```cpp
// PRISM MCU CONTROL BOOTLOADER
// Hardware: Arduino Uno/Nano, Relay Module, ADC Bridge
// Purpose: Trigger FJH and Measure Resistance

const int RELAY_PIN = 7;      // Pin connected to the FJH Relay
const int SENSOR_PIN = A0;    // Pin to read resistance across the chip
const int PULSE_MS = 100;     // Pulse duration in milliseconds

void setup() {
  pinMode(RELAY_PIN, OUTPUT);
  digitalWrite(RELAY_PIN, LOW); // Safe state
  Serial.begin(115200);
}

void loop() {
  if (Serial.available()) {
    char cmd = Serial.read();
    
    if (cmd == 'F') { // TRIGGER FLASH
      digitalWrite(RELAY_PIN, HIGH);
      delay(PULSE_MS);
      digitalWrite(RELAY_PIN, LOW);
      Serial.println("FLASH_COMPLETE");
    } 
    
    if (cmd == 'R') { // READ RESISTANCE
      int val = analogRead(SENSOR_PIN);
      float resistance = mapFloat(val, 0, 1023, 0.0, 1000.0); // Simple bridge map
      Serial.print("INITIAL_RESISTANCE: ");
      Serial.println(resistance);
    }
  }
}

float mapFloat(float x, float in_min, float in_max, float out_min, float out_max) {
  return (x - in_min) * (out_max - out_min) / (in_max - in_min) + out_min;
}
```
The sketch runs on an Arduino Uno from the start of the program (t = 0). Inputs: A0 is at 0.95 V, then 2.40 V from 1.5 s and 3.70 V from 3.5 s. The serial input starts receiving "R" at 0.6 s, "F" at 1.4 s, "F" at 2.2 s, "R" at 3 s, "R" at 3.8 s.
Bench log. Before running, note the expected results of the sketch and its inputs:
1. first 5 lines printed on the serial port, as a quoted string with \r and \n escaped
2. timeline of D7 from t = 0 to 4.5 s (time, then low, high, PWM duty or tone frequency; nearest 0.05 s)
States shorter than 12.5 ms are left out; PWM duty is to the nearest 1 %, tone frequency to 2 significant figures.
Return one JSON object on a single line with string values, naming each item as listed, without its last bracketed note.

{"first 5 lines printed on the serial port, as a quoted string with \\r and \\n escaped": "\"INITIAL_RESISTANCE: 189.64\\r\\nFLASH_COMPLETE\\r\\nFLASH_COMPLETE\\r\\nINITIAL_RESISTANCE: 479.96\\r\\nINITIAL_RESISTANCE: 739.98\\r\\n\"", "timeline of D7 from t = 0 to 4.5 s": "0 s low; 1.4 s high; 1.5 s low; 2.2 s high; 2.3 s low"}
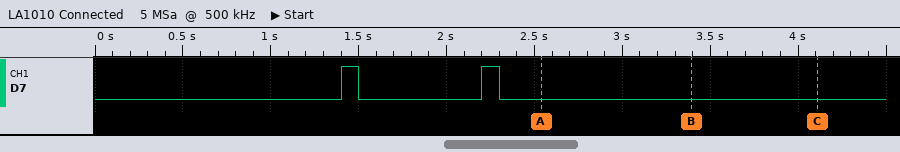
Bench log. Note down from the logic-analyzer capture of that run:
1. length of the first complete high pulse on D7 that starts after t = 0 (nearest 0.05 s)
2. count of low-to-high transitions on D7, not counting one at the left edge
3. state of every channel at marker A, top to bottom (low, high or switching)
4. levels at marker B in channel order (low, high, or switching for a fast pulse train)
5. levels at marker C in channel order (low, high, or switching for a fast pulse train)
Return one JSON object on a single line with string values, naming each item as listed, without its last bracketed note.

{"length of the first complete high pulse on D7 that starts after t = 0": "0.10 s", "count of low-to-high transitions on D7, not counting one at the left edge": "2", "state of every channel at marker A, top to bottom": "D7 low", "levels at marker B in channel order": "D7 low", "levels at marker C in channel order": "D7 low"}
